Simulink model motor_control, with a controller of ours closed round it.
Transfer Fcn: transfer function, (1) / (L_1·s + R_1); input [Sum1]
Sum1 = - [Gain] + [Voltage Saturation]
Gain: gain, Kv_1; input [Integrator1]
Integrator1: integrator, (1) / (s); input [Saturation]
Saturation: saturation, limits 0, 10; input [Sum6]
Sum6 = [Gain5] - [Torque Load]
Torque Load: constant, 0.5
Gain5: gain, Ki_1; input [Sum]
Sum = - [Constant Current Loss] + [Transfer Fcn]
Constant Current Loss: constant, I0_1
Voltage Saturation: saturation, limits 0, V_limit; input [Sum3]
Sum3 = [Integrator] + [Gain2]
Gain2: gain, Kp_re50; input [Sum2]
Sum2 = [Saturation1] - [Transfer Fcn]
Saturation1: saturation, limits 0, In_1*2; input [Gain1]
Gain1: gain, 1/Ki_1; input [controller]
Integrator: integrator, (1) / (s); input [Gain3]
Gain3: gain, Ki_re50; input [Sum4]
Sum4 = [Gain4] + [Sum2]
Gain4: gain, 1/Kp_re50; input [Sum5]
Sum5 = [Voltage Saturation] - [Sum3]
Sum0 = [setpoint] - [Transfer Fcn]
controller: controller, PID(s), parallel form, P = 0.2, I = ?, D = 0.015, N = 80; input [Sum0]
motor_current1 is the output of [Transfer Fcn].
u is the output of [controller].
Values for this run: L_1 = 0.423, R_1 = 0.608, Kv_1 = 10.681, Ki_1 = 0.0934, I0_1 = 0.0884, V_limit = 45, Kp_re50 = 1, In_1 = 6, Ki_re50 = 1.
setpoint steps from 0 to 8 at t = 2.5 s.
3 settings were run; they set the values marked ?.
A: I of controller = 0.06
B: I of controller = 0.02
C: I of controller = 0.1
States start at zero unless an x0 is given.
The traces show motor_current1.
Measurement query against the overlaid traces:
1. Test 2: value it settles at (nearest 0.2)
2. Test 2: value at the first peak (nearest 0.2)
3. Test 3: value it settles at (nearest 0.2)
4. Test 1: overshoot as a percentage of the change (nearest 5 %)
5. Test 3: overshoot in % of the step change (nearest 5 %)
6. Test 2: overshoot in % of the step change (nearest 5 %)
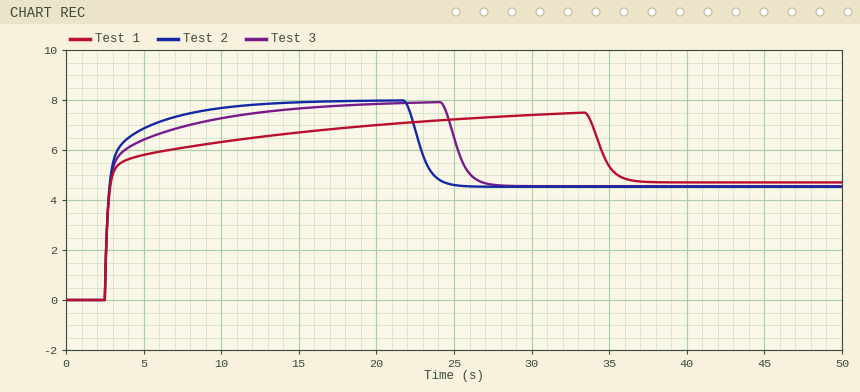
4.6
8.0
4.6
60 %
75 %
75 %
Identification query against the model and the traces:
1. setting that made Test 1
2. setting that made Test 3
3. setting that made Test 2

B
A
C
